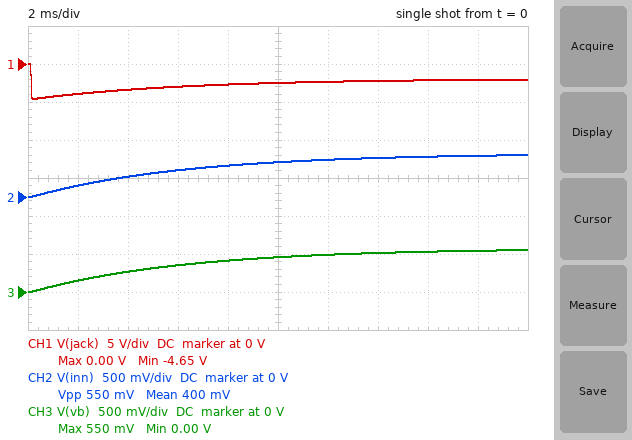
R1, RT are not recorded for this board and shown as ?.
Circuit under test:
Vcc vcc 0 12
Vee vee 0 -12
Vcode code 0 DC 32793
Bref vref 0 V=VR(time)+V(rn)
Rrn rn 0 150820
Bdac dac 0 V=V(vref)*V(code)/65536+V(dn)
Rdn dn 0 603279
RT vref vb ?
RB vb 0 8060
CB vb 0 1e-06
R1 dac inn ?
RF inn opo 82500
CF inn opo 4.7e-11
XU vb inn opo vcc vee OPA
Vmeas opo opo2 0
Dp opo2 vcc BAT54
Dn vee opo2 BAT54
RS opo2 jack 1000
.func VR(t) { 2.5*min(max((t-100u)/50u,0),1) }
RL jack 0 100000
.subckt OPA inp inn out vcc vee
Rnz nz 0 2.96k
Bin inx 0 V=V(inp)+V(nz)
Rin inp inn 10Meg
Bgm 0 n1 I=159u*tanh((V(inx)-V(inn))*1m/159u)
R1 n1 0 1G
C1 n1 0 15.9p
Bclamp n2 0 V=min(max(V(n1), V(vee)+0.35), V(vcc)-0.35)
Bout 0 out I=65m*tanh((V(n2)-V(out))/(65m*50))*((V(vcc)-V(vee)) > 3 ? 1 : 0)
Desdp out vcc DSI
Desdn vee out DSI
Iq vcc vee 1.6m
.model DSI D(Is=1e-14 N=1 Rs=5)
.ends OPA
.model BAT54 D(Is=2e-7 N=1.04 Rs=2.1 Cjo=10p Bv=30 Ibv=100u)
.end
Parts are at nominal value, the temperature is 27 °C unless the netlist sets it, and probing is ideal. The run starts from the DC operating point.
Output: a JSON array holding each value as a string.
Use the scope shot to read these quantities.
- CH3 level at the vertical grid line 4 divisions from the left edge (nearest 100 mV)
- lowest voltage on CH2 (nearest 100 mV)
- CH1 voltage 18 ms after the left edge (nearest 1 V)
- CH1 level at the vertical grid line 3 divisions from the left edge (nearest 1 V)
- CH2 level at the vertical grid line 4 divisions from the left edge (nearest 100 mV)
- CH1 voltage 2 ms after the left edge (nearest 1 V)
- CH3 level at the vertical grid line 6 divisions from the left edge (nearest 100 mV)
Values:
["400 mV", "0 V", "-2 V", "-3 V", "400 mV", "-4 V", "500 mV"]
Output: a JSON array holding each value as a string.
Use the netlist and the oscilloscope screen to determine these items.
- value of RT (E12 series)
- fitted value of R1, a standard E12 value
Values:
["27 kΩ", "22 kΩ"]
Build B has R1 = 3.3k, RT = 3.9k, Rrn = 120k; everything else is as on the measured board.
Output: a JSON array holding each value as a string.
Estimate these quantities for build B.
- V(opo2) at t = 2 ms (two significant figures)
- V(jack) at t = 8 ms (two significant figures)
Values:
["-12 V", "10 V"]
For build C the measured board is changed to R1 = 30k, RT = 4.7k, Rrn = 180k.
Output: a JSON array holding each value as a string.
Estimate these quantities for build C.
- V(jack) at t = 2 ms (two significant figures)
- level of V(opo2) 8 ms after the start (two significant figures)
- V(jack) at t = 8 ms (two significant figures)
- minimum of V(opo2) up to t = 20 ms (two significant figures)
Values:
["-660 mV", "2.1 V", "2.0 V", "-3.4 V"]
